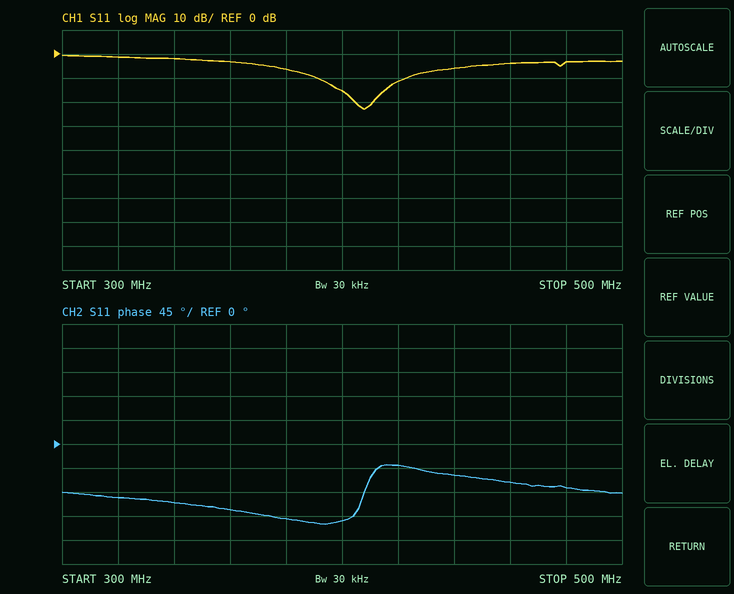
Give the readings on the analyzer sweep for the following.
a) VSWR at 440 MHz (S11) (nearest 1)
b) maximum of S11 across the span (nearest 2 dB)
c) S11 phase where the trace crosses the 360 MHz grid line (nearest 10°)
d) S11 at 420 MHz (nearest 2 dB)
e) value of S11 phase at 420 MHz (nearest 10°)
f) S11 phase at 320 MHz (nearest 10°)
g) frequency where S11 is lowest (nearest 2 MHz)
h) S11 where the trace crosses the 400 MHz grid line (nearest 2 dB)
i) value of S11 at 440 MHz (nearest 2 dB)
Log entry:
3
0 dB
-120°
-12 dB
-40°
-100°
408 MHz
-16 dB
-6 dB
